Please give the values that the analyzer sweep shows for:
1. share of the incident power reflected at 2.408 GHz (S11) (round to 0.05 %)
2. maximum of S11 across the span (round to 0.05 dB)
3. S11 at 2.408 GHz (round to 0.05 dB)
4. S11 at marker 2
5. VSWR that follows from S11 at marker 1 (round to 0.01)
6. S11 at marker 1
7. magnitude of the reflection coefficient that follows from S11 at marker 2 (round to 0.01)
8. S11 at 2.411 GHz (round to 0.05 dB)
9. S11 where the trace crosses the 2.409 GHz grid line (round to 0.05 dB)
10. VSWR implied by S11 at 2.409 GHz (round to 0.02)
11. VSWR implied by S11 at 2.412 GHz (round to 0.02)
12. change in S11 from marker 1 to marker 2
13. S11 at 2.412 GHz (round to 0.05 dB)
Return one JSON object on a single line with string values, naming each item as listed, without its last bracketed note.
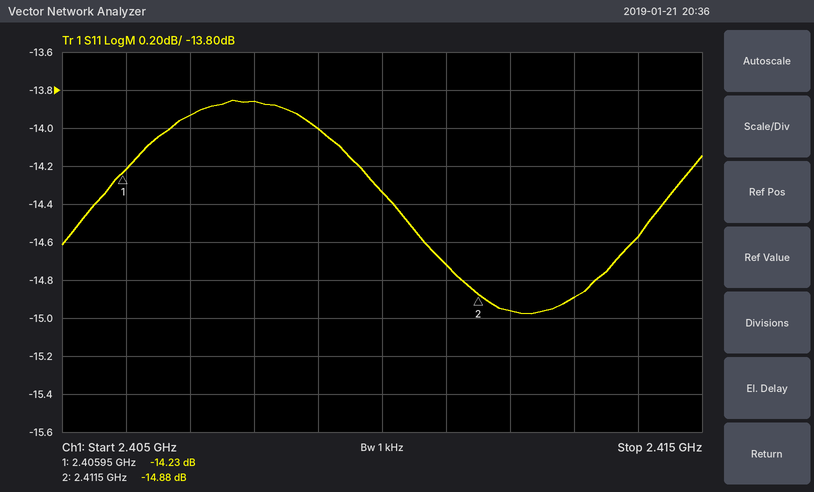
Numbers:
{"share of the incident power reflected at 2.408 GHz (S11)": "4.10 %", "maximum of S11 across the span": "-13.85 dB", "S11 at 2.408 GHz": "-13.85 dB", "S11 at marker 2": "-14.88 dB", "VSWR that follows from S11 at marker 1": "1.48", "S11 at marker 1": "-14.23 dB", "magnitude of the reflection coefficient that follows from S11 at marker 2": "0.18", "S11 at 2.411 GHz": "-14.70 dB", "S11 where the trace crosses the 2.409 GHz grid line": "-14.00 dB", "VSWR implied by S11 at 2.409 GHz": "1.50", "VSWR implied by S11 at 2.412 GHz": "1.44", "change in S11 from marker 1 to marker 2": "-0.65 dB", "S11 at 2.412 GHz": "-14.95 dB"}
